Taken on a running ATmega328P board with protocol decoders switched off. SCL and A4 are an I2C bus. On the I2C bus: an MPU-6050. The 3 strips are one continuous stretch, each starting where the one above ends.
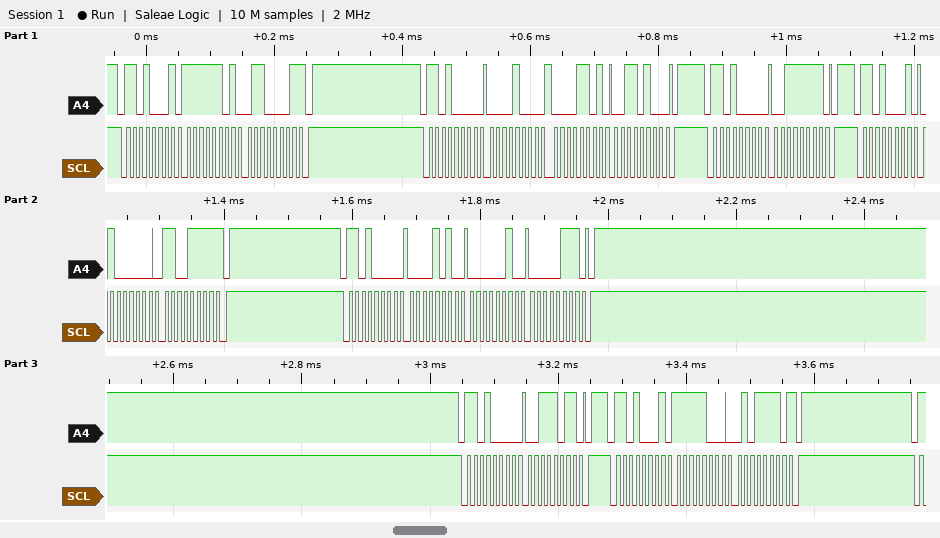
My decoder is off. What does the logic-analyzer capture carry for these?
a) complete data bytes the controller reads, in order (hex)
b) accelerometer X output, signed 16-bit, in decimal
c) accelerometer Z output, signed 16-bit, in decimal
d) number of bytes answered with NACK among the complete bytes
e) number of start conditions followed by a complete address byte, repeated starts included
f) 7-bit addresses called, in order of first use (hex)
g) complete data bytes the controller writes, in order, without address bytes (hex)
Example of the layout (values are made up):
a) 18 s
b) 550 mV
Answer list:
a) FD 61 40 CF F8 5E
b) -1954
c) 16591
d) 3
e) 7
f) 0x68
g) 08 0D 34 3F 0A 02 07 3B
